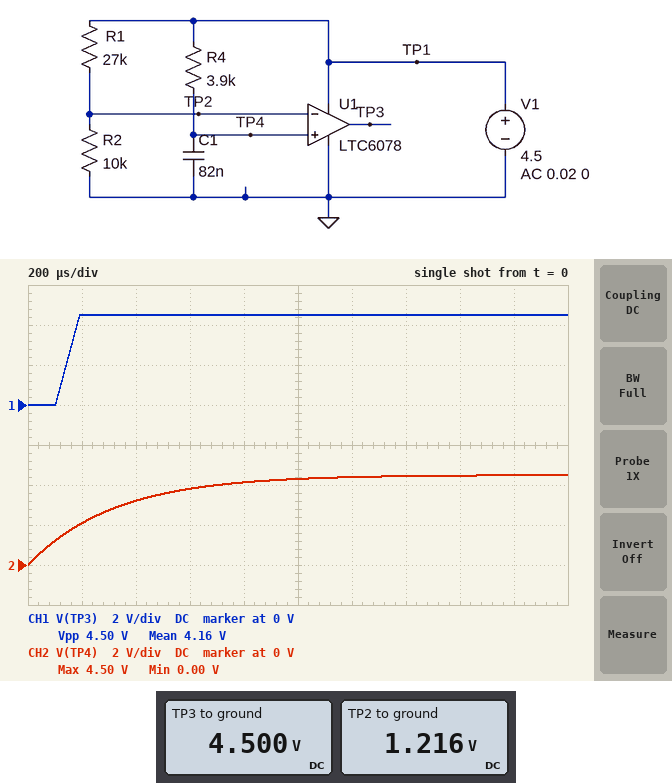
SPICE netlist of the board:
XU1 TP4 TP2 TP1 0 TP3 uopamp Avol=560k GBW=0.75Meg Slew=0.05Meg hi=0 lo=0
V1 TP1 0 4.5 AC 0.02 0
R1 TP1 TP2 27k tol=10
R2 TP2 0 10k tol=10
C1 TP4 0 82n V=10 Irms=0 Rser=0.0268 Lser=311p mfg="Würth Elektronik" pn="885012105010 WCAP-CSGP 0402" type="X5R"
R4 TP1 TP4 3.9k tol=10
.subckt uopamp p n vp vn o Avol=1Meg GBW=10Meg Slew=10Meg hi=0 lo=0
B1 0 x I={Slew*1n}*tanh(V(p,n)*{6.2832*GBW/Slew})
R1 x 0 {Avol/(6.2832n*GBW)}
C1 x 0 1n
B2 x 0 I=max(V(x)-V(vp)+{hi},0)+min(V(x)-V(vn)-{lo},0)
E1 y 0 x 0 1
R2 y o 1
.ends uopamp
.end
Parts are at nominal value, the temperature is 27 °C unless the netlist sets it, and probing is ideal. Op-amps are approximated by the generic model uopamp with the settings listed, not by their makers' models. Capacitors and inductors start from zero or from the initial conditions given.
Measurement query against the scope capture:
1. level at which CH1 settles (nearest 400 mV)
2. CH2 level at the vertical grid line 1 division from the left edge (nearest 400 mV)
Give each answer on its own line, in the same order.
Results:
4.4 V
2.0 V
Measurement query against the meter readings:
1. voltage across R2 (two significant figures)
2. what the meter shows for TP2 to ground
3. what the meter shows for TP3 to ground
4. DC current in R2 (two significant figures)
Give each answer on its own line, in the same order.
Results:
1.2 V
1.216 V
4.500 V
120 µA
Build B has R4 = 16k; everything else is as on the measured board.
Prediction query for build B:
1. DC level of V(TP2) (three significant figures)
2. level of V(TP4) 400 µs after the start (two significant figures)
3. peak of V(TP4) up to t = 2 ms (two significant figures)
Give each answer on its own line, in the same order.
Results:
1.22 V
1.2 V
3.5 V
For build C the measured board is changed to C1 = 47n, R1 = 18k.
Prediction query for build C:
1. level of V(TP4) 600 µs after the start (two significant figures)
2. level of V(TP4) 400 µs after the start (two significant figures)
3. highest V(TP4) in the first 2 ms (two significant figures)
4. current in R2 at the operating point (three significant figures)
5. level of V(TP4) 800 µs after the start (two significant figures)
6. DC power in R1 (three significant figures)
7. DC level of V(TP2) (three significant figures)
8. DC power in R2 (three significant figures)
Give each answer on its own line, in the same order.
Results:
4.3 V
4.0 V
4.5 V
161 µA
4.4 V
465 µW
1.61 V
258 µW
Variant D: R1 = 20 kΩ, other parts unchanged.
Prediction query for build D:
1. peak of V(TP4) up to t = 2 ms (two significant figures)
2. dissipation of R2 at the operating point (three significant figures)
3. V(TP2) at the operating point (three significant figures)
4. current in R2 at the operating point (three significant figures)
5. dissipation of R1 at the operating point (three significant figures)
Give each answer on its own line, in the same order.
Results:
4.5 V
225 µW
1.50 V
150 µA
450 µW
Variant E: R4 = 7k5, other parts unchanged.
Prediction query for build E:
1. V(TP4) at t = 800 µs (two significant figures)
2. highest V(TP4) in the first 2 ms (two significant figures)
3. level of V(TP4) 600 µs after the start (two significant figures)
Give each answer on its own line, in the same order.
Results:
3.3 V
4.3 V
2.8 V
